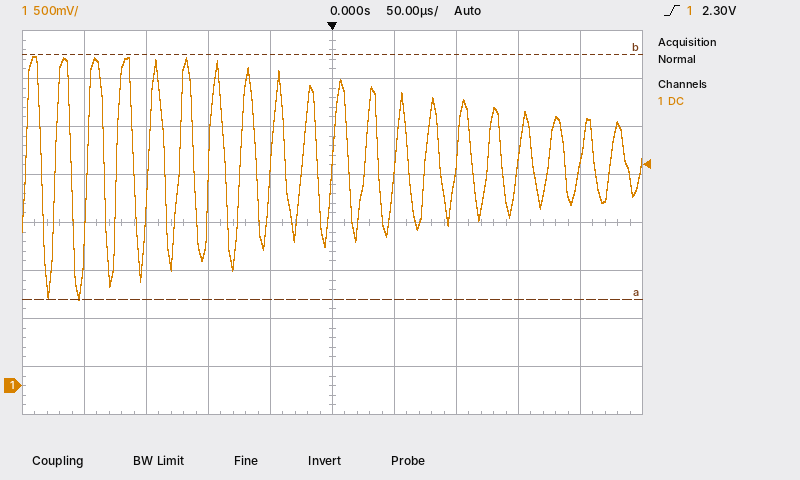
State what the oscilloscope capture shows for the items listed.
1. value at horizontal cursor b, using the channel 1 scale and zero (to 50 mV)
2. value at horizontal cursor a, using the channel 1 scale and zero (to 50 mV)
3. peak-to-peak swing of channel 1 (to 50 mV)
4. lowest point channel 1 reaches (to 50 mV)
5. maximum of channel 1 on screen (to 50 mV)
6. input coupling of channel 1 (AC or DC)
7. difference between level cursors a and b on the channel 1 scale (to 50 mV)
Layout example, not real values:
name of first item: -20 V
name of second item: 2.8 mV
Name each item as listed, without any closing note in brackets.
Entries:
value at horizontal cursor b, using the channel 1 scale and zero: 3.45 V
value at horizontal cursor a, using the channel 1 scale and zero: 900 mV
peak-to-peak swing of channel 1: 2.55 V
lowest point channel 1 reaches: 900 mV
maximum of channel 1 on screen: 3.45 V
input coupling of channel 1: DC
difference between level cursors a and b on the channel 1 scale: 2.55 V
